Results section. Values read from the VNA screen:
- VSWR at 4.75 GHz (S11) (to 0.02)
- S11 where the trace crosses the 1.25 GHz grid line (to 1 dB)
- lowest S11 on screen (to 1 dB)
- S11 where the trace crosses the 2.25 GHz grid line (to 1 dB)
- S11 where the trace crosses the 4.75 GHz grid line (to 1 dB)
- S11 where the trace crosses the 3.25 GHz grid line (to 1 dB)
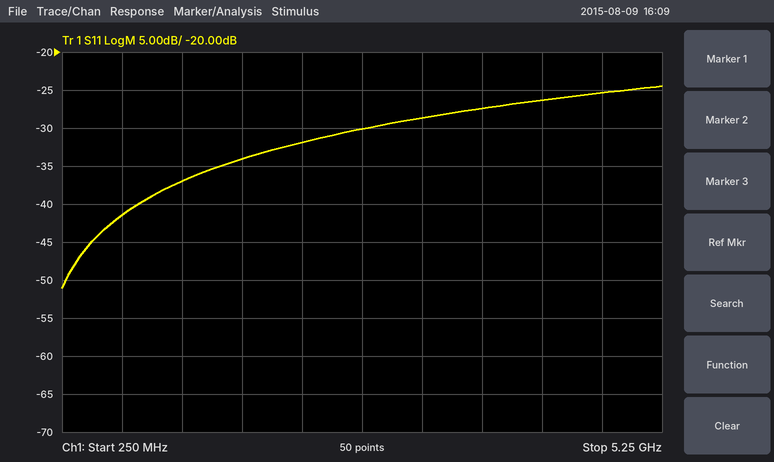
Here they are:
1.12
-37 dB
-51 dB
-32 dB
-25 dB
-29 dB
